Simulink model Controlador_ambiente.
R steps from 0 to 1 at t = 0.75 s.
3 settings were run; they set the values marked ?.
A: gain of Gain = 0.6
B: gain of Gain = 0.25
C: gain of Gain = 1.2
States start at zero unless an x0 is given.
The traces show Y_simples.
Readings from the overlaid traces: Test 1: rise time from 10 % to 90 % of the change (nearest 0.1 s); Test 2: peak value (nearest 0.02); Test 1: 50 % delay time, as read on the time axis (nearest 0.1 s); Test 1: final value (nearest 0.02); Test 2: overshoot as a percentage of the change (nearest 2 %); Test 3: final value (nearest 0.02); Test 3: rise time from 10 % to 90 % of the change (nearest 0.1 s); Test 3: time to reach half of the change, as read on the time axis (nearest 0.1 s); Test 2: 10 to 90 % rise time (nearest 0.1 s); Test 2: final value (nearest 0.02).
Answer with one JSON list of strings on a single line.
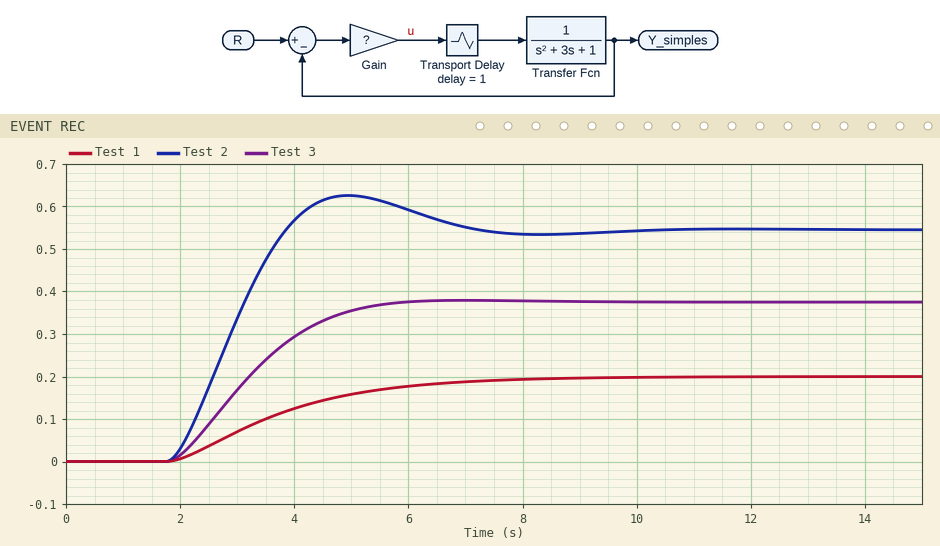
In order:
["4.0 s", "0.62", "3.5 s", "0.20", "14 %", "0.38", "2.4 s", "3.1 s", "1.5 s", "0.54"]
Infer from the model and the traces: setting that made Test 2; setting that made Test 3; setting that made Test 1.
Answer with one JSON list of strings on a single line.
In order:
["C", "A", "B"]
